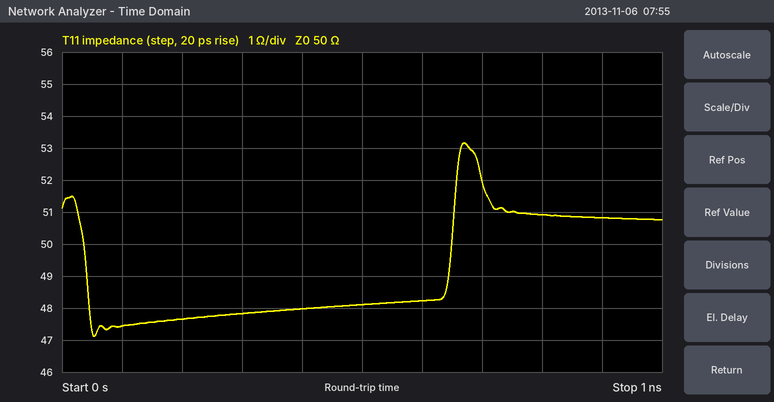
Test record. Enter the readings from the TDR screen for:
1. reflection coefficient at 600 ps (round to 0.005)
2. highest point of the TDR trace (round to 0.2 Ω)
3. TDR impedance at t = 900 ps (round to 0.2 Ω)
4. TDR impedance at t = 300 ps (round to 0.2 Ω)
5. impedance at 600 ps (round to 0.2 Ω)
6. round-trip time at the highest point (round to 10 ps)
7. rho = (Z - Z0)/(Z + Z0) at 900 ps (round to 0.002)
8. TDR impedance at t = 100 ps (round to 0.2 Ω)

-0.020
53.2 Ω
50.8 Ω
47.8 Ω
48.2 Ω
670 ps
+0.008
47.4 Ω
